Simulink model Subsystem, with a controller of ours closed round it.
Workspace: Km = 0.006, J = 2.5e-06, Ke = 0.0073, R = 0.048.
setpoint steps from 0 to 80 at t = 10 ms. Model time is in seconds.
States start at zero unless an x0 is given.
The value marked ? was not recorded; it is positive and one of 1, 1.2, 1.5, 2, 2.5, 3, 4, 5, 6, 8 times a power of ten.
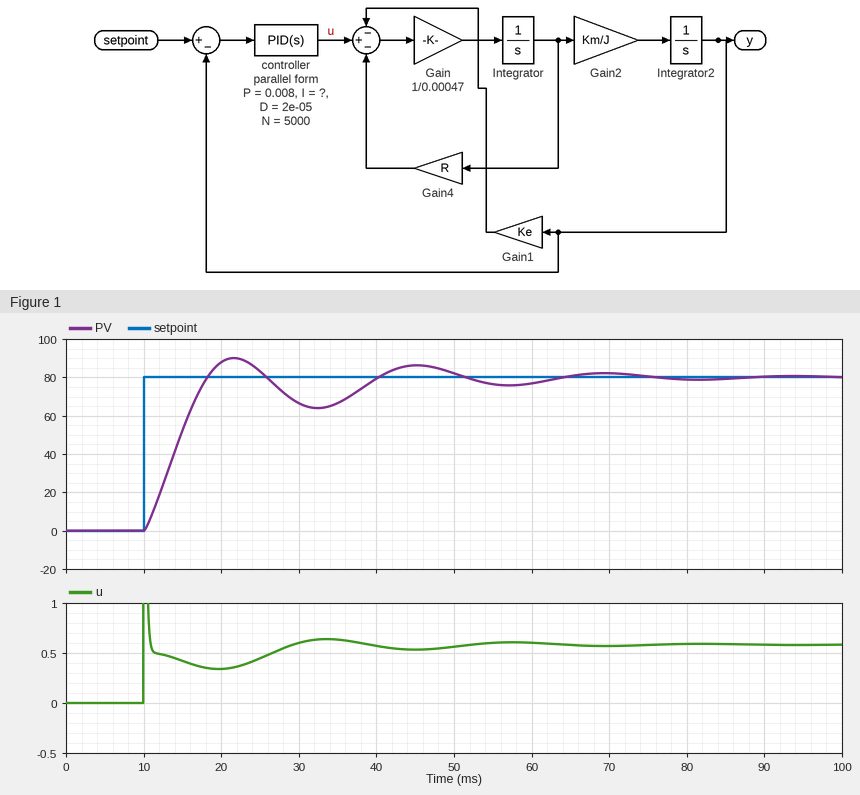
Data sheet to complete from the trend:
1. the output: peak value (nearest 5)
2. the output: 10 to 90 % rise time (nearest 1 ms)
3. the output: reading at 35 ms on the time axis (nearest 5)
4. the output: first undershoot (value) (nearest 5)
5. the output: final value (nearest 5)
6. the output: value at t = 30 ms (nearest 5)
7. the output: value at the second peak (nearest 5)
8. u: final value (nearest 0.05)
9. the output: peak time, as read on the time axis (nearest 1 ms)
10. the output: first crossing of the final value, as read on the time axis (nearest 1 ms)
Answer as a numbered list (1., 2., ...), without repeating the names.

1. 90
2. 6 ms
3. 65
4. 65
5. 80
6. 65
7. 85
8. 0.60
9. 22 ms
10. 18 ms
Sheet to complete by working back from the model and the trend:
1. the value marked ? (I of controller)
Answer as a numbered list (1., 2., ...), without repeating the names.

1. 1.5
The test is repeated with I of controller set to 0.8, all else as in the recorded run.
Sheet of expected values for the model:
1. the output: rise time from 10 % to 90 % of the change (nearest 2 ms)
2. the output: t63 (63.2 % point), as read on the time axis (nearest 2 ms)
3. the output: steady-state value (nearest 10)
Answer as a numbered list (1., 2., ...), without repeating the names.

1. 8 ms
2. 16 ms
3. 80
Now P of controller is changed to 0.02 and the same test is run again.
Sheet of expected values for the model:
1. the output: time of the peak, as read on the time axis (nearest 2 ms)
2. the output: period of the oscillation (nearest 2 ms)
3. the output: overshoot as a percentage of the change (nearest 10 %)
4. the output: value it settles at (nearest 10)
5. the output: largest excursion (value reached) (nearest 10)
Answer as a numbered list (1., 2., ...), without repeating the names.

1. 18 ms
2. 18 ms
3. 20 %
4. 80
5. 100
